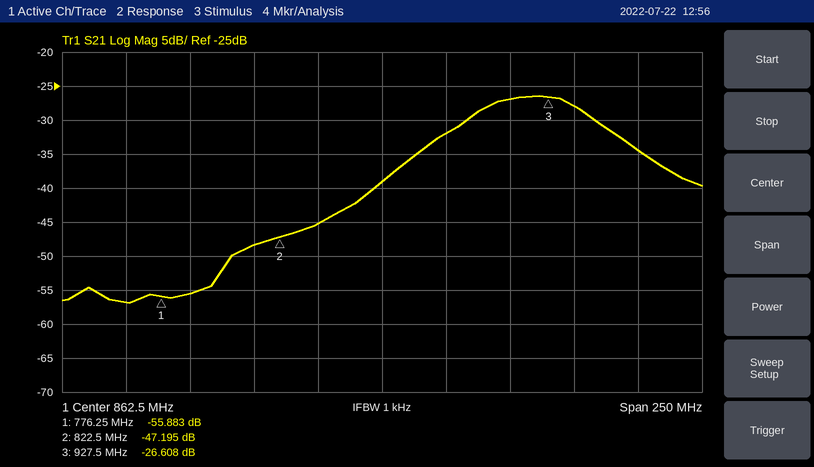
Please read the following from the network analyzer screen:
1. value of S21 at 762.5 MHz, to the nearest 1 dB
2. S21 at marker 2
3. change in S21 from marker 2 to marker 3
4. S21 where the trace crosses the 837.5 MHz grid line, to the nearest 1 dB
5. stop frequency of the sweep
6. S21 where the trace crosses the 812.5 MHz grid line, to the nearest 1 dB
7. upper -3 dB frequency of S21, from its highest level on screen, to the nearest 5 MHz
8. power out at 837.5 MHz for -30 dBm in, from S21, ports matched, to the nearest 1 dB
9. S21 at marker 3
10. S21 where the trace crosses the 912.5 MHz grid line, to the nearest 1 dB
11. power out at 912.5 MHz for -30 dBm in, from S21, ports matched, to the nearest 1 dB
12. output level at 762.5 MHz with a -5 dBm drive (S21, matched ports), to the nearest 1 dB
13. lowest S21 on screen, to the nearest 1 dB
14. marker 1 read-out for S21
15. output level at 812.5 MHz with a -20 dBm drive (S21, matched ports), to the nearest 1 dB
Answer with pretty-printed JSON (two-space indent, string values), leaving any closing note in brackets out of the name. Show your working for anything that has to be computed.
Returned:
{
  "value of S21 at 762.5 MHz, to the nearest 1 dB": "-57 dB",
  "S21 at marker 2": "-47.195 dB",
  "change in S21 from marker 2 to marker 3": "-26.608 − (-47.195) = 20.587 dB",
  "S21 where the trace crosses the 837.5 MHz grid line, to the nearest 1 dB": "-45 dB",
  "stop frequency of the sweep": "987.5 MHz",
  "S21 where the trace crosses the 812.5 MHz grid line, to the nearest 1 dB": "-48 dB",
  "upper -3 dB frequency of S21, from its highest level on screen, to the nearest 5 MHz": "945 MHz",
  "power out at 837.5 MHz for -30 dBm in, from S21, ports matched, to the nearest 1 dB": "-30 dBm + (-45 dB) = -75 dBm",
  "S21 at marker 3": "-26.608 dB",
  "S21 where the trace crosses the 912.5 MHz grid line, to the nearest 1 dB": "-27 dB",
  "power out at 912.5 MHz for -30 dBm in, from S21, ports matched, to the nearest 1 dB": "-30 dBm + (-27 dB) = -57 dBm",
  "output level at 762.5 MHz with a -5 dBm drive (S21, matched ports), to the nearest 1 dB": "-5 dBm + (-57 dB) = -62 dBm",
  "lowest S21 on screen, to the nearest 1 dB": "-57 dB",
  "marker 1 read-out for S21": "-55.883 dB",
  "output level at 812.5 MHz with a -20 dBm drive (S21, matched ports), to the nearest 1 dB": "-20 dBm + (-48 dB) = -68 dBm"
}
